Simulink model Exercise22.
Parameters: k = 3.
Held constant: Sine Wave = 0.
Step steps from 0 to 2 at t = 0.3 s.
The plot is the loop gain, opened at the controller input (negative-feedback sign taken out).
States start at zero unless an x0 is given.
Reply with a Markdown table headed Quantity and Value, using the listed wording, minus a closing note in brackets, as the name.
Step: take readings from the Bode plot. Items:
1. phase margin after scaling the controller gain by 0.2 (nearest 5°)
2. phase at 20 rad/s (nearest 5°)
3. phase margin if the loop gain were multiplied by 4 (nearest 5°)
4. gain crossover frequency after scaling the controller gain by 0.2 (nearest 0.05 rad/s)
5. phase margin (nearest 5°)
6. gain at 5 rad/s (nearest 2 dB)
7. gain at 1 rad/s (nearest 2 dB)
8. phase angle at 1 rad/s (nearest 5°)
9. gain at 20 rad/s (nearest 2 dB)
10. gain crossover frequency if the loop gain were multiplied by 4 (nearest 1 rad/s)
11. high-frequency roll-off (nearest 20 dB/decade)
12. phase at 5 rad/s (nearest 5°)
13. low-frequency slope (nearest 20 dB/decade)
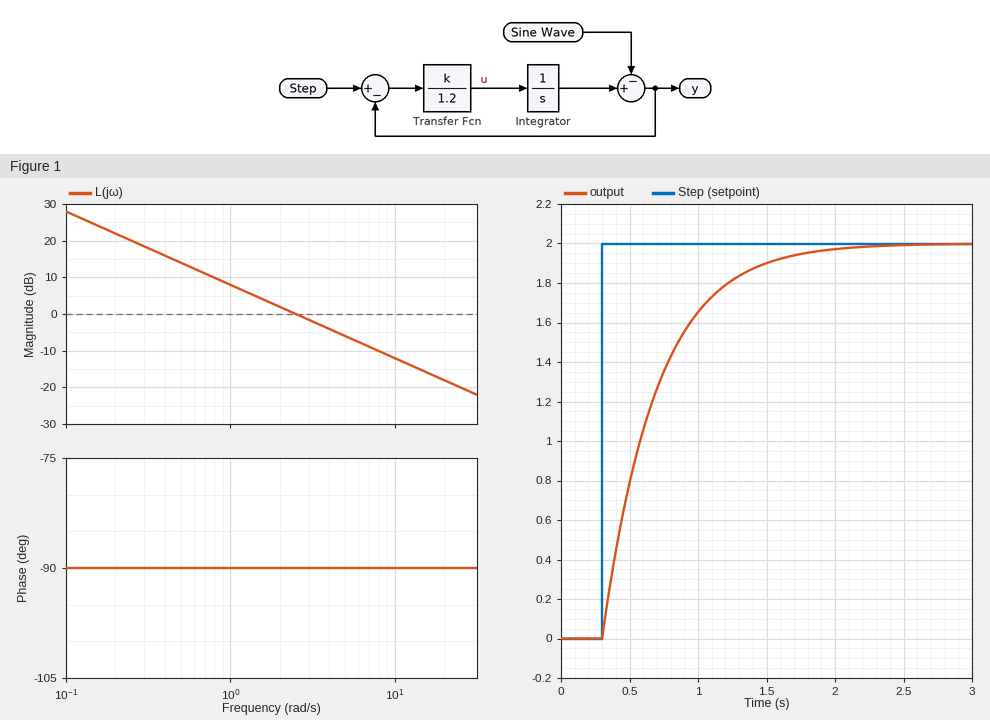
| Quantity | Value |
|---|---|
| phase margin after scaling the controller gain by 0.2 | 90° |
| phase at 20 rad/s | -90° |
| phase margin if the loop gain were multiplied by 4 | 90° |
| gain crossover frequency after scaling the controller gain by 0.2 | 0.50 rad/s |
| phase margin | 90° |
| gain at 5 rad/s | -6 dB |
| gain at 1 rad/s | 8 dB |
| phase angle at 1 rad/s | -90° |
| gain at 20 rad/s | -18 dB |
| gain crossover frequency if the loop gain were multiplied by 4 | 10 rad/s |
| high-frequency roll-off | -20 dB/decade |
| phase at 5 rad/s | -90° |
| low-frequency slope | -20 dB/decade |
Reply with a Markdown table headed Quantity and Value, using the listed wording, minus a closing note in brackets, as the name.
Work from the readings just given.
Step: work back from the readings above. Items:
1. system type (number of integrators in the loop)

| Quantity | Value |
|---|---|
| system type | 1 |
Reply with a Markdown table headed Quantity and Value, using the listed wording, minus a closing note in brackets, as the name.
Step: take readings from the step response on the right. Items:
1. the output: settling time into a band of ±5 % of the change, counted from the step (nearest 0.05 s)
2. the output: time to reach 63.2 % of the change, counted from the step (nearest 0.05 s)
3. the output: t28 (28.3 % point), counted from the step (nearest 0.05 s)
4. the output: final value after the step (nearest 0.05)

| Quantity | Value |
|---|---|
| the output: settling time into a band of ±5 % of the change, counted from the step | 1.20 s |
| the output: time to reach 63.2 % of the change, counted from the step | 0.40 s |
| the output: t28 (28.3 % point), counted from the step | 0.15 s |
| the output: final value after the step | 2.00 |
